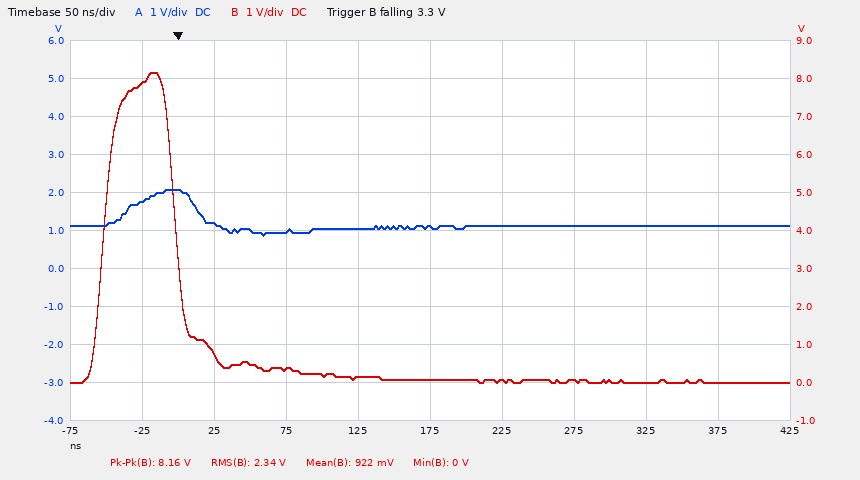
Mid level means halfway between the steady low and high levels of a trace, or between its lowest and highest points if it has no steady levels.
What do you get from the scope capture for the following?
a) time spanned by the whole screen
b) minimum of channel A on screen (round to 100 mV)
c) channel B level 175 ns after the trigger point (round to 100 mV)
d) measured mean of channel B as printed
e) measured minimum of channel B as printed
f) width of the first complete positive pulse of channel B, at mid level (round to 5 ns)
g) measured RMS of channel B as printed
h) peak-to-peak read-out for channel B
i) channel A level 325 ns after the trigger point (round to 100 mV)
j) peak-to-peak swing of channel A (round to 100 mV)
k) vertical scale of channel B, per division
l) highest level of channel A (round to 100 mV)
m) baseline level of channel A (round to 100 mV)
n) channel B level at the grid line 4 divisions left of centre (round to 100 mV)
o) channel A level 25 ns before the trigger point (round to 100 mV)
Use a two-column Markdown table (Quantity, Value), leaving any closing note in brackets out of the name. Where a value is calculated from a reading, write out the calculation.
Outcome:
| Quantity | Value |
|---|---|
| time spanned by the whole screen | 500 ns |
| minimum of channel A on screen | 900 mV |
| channel B level 175 ns after the trigger point | 100 mV |
| measured mean of channel B as printed | 922 mV |
| measured minimum of channel B as printed | 0 V |
| width of the first complete positive pulse of channel B, at mid level | 50 ns |
| measured RMS of channel B as printed | 2.34 V |
| peak-to-peak read-out for channel B | 8.16 V |
| channel A level 325 ns after the trigger point | 1.1 V |
| peak-to-peak swing of channel A | 2.1 V − (900 mV) = 1.2 V |
| vertical scale of channel B, per division | 1 V |
| highest level of channel A | 2.1 V |
| baseline level of channel A | 1.1 V |
| channel B level at the grid line 4 divisions left of centre | 7.9 V |
| channel A level 25 ns before the trigger point | 1.8 V |
